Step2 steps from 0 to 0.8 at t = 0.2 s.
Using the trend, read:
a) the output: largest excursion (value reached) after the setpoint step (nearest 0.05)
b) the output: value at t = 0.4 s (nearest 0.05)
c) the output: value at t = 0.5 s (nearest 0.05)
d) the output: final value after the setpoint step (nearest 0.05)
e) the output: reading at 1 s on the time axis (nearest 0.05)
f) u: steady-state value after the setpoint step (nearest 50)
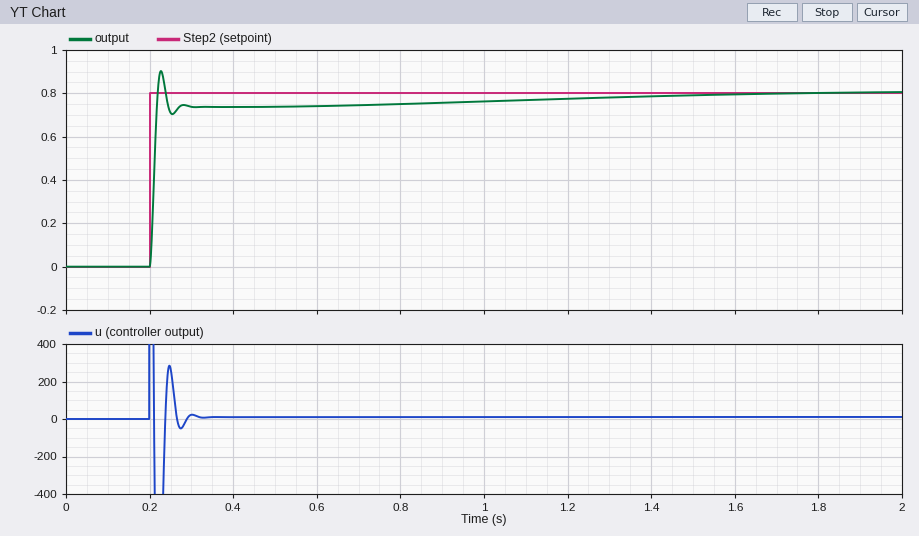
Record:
0.90
0.75
0.75
0.80
0.75
0
